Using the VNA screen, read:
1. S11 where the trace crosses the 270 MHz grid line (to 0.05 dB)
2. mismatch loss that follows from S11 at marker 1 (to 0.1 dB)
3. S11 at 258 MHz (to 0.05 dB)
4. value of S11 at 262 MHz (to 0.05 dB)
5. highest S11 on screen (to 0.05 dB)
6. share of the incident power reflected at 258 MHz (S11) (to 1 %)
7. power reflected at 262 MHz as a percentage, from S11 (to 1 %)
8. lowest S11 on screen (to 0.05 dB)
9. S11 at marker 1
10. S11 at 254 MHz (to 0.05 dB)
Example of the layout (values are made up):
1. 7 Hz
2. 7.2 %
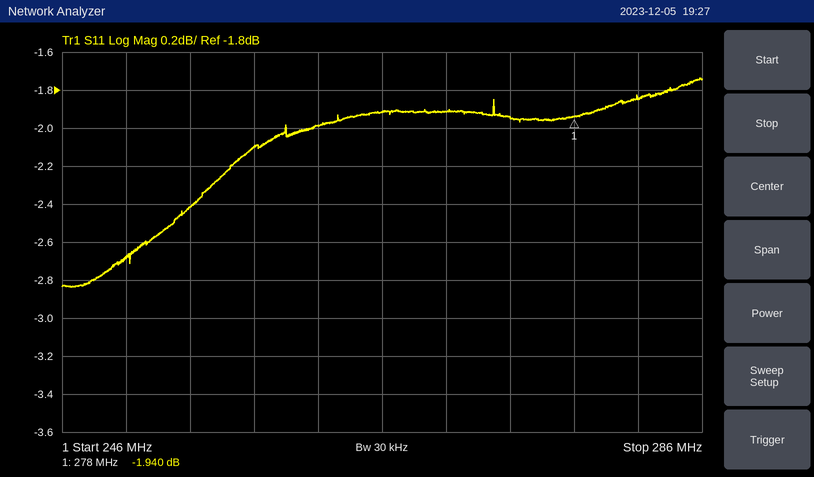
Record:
1. -1.90 dB
2. 4.4 dB
3. -2.10 dB
4. -2.00 dB
5. -1.75 dB
6. 62 %
7. 63 %
8. -2.85 dB
9. -1.940 dB
10. -2.40 dB
